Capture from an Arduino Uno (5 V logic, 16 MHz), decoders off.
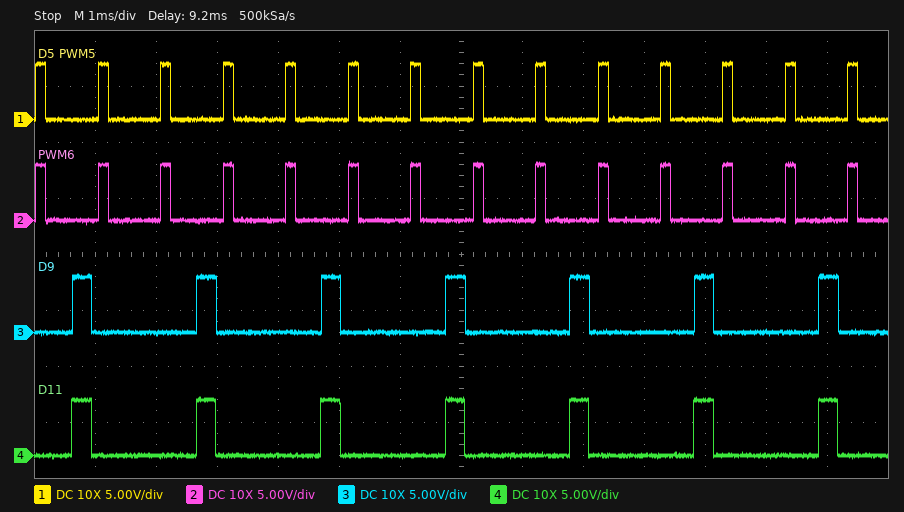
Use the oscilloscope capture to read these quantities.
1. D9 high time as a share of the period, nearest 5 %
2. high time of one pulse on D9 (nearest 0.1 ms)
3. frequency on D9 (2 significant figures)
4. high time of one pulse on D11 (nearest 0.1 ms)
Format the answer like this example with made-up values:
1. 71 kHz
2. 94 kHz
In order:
1. 15 %
2. 0.3 ms
3. 490 Hz
4. 0.3 ms
